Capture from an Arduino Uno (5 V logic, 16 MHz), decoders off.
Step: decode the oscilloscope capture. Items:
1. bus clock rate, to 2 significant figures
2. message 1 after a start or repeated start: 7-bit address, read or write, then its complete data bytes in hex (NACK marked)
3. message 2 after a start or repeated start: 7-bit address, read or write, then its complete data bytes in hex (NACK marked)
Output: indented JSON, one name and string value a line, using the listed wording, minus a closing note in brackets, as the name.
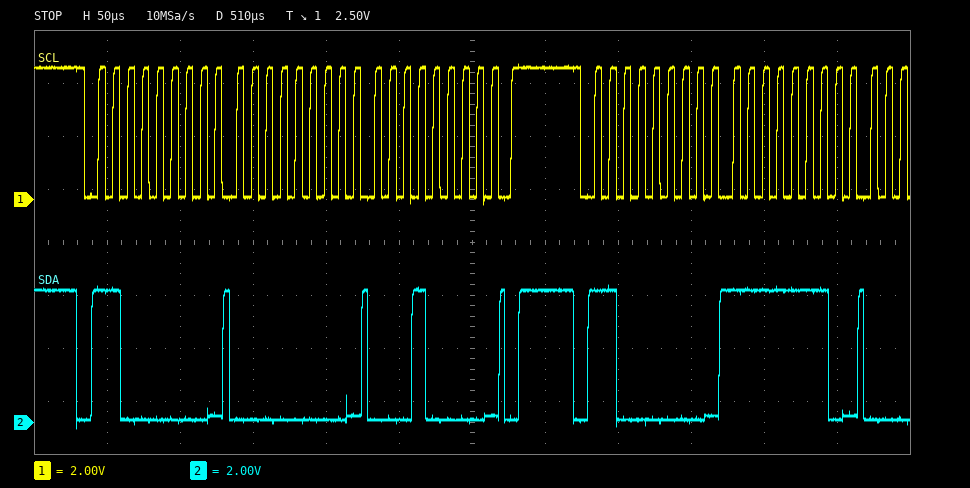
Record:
{
  "bus clock rate, to 2 significant figures": "100 kHz",
  "message 1 after a start or repeated start: 7-bit address, read or write, then its complete data bytes in hex": "0x60 write: 00 10",
  "message 2 after a start or repeated start: 7-bit address, read or write, then its complete data bytes in hex": "0x60 write: FE"
}
